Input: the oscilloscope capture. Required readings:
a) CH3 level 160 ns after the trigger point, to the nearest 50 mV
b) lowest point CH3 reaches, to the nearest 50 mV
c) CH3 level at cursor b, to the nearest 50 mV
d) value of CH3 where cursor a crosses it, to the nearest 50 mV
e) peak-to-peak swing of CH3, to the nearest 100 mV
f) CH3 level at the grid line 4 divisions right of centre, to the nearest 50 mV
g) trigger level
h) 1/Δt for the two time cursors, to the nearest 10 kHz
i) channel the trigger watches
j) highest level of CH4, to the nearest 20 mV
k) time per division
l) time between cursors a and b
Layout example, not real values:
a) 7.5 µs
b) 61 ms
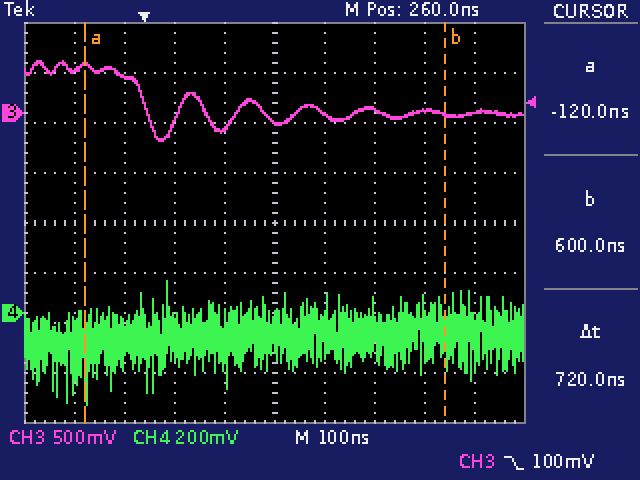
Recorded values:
a) -150 mV
b) -300 mV
c) 0 mV
d) 450 mV
e) 800 mV
f) 0 mV
g) 100 mV
h) 1.39 MHz
i) CH3
j) 120 mV
k) 100 ns
l) 720 ns
